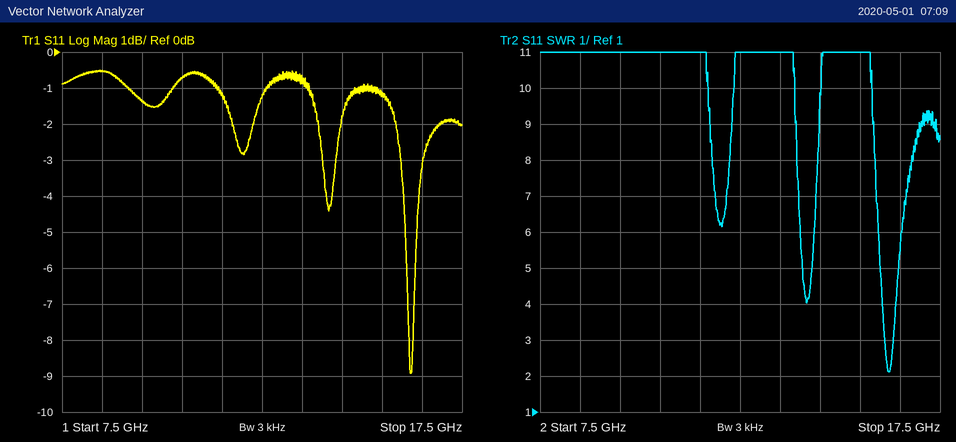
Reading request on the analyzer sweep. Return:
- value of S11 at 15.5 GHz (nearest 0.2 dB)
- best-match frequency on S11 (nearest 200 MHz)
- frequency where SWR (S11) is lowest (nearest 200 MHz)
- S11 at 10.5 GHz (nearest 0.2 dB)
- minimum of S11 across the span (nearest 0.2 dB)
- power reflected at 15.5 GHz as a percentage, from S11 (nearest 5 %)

-1.2 dB
16.2 GHz
16.2 GHz
-0.8 dB
-9.0 dB
75 %
